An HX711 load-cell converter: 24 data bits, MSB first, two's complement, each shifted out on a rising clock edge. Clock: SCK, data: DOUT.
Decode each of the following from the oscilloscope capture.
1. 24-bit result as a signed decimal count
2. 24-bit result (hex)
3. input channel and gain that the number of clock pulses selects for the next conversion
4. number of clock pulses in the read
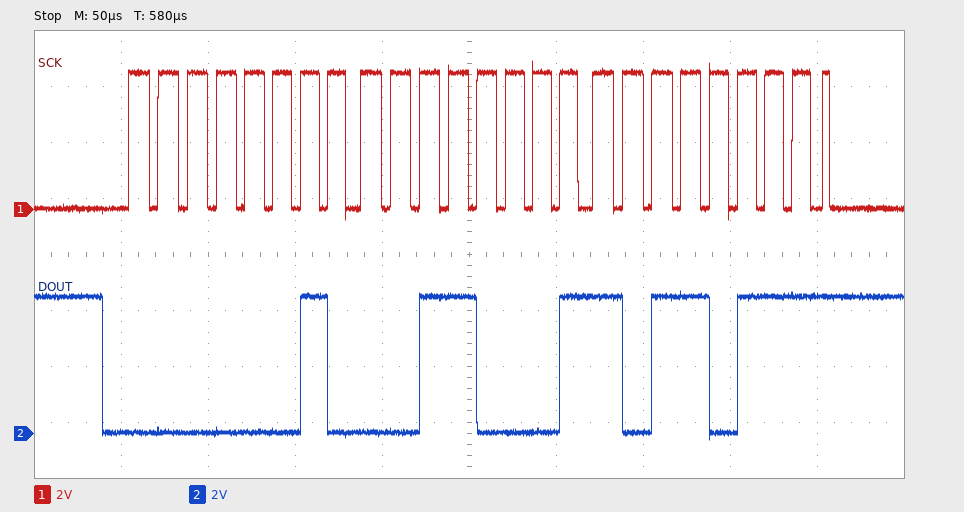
143799
0x0231B7
channel A, gain 128
25
